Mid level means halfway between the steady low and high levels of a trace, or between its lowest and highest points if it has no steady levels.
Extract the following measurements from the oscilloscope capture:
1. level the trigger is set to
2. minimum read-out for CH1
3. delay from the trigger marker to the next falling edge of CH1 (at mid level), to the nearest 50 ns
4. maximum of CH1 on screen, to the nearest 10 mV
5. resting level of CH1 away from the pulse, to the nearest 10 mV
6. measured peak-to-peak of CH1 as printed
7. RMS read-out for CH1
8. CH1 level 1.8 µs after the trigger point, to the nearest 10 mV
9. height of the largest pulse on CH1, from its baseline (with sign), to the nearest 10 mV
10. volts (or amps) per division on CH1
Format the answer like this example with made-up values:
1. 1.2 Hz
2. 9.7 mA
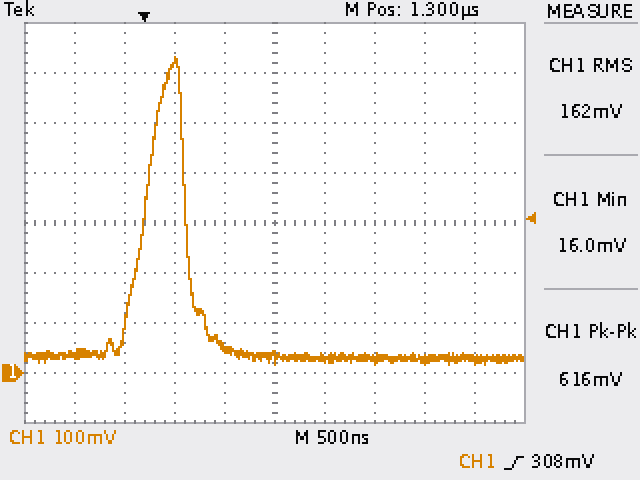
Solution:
1. 308 mV
2. 16.0 mV
3. 400 ns
4. 630 mV
5. 30 mV
6. 616 mV
7. 162 mV
8. 30 mV
9. +600 mV
10. 100 mV
